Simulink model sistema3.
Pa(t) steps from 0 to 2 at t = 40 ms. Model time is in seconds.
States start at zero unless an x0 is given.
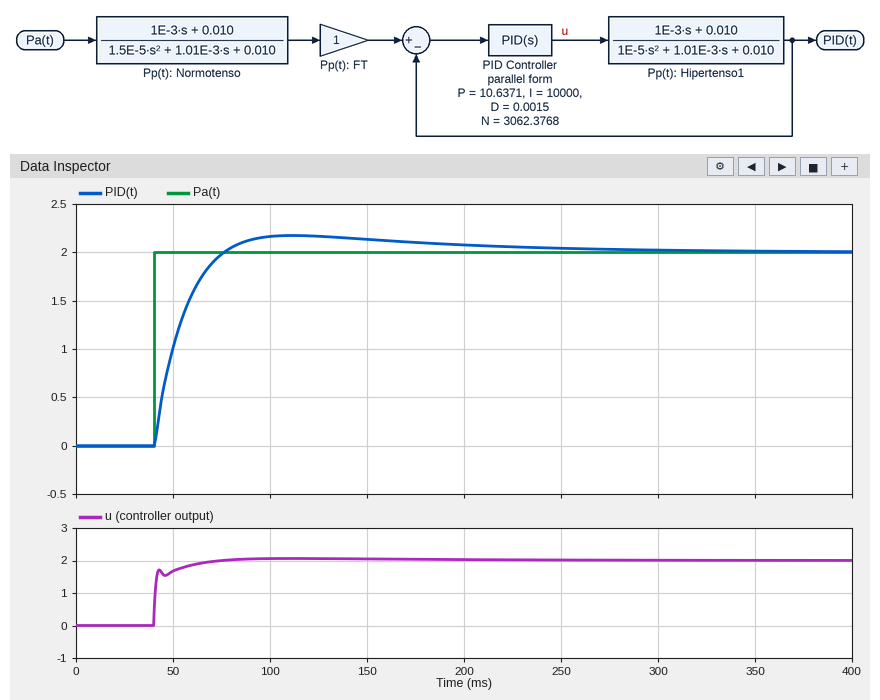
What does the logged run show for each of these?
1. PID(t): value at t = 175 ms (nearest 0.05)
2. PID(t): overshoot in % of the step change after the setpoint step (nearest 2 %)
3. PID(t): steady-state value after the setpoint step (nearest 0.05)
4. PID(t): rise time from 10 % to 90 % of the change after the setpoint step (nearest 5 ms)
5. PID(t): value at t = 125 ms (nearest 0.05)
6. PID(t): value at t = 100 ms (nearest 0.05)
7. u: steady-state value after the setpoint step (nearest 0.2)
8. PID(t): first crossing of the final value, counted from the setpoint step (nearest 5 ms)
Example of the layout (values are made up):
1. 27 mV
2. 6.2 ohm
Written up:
1. 2.10
2. 8 %
3. 2.00
4. 25 ms
5. 2.15
6. 2.15
7. 2.0
8. 35 ms
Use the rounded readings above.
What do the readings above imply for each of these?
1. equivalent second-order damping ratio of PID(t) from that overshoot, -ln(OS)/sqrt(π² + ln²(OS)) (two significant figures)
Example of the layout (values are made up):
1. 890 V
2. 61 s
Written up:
1. 0.63
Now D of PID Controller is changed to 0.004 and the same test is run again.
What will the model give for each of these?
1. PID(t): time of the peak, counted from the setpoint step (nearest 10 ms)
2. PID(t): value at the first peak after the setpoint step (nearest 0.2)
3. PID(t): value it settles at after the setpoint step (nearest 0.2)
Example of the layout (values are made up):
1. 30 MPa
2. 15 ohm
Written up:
1. 70 ms
2. 2.2
3. 2.0
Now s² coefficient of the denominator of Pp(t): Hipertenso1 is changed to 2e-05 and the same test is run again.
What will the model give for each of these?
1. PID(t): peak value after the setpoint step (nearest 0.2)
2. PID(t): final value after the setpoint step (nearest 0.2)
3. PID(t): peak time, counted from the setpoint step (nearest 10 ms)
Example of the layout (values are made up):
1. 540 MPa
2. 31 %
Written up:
1. 2.2
2. 2.0
3. 70 ms
